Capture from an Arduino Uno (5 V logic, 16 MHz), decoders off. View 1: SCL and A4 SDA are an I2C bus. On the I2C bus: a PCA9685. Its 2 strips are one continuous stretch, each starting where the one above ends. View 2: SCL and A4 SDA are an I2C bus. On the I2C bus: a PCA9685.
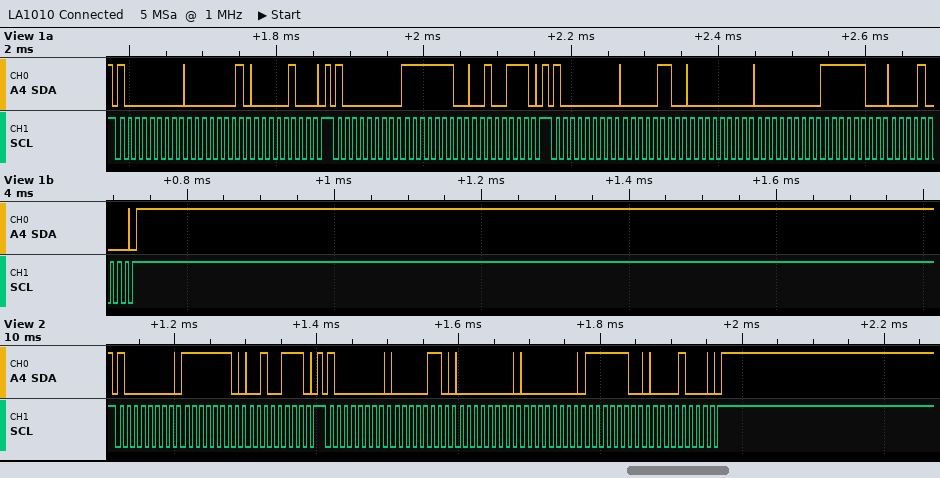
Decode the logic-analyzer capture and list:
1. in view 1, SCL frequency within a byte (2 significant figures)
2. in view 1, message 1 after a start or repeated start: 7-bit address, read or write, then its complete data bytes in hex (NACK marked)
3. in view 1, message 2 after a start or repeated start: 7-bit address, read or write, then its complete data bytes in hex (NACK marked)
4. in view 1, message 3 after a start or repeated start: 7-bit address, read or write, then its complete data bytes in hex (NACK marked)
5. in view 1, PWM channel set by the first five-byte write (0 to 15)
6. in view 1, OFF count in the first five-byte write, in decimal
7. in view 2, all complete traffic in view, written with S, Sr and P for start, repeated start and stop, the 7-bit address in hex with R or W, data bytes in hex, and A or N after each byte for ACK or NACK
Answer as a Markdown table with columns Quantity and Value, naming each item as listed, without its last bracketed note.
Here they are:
| Quantity | Value |
|---|---|
| in view 1, SCL frequency within a byte | 100 kHz |
| in view 1, message 1 after a start or repeated start: 7-bit address, read or write, then its complete data bytes in hex | 0x40 write: 01 04 |
| in view 1, message 2 after a start or repeated start: 7-bit address, read or write, then its complete data bytes in hex | 0x40 write: FE 27 |
| in view 1, message 3 after a start or repeated start: 7-bit address, read or write, then its complete data bytes in hex | 0x40 write: 06 00 00 FC 08 |
| in view 1, PWM channel set by the first five-byte write | 0 |
| in view 1, OFF count in the first five-byte write, in decimal | 2300 |
| in view 2, all complete traffic in view, written with S, Sr and P for start, repeated start and stop, the 7-bit address in hex with R or W, data bytes in hex, and A or N after each byte for ACK or NACK | S 40W A FE A 27 A P S 40W A 06 A 00 A 00 A FC A 08 A P |
